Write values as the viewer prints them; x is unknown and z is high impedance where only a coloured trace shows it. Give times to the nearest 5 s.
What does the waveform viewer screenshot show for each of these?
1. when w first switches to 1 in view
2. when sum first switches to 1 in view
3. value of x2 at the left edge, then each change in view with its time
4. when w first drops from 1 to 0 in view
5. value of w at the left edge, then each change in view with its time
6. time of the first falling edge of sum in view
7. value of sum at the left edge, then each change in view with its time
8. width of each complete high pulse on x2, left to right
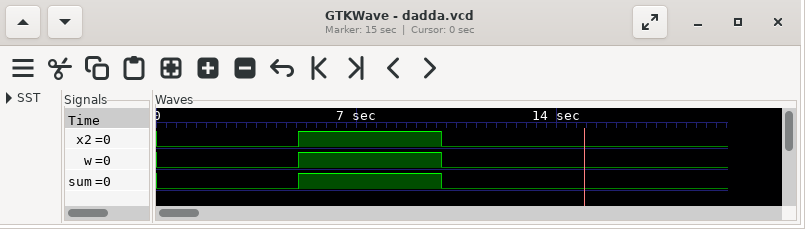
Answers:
5 s
5 s
0, 1 at 5 s, 0 at 10 s
10 s
0, 1 at 5 s, 0 at 10 s
10 s
0, 1 at 5 s, 0 at 10 s
5 s
